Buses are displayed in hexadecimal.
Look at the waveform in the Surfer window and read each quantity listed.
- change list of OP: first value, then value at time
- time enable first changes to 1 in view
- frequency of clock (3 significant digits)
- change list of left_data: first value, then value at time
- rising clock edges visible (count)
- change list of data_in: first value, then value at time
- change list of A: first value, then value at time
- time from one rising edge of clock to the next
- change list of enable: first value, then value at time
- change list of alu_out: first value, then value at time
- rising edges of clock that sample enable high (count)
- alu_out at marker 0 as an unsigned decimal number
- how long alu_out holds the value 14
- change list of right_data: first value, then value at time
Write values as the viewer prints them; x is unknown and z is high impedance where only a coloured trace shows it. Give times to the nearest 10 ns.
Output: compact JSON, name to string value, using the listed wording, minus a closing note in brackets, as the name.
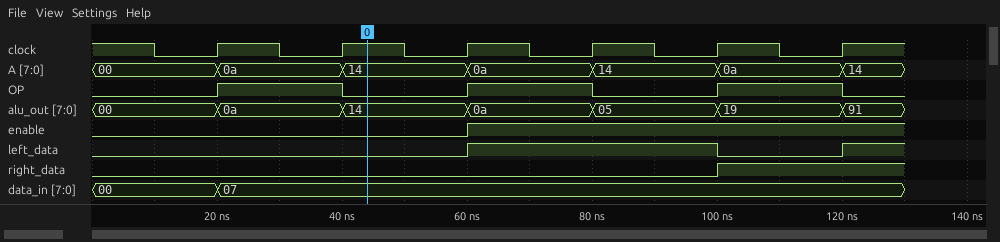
{"change list of OP: first value, then value at time": "0, 1 at 20 ns, 0 at 40 ns, 1 at 60 ns, 0 at 80 ns, 1 at 100 ns, 0 at 120 ns", "time enable first changes to 1 in view": "60 ns", "frequency of clock": "50.0 MHz", "change list of left_data: first value, then value at time": "0, 1 at 60 ns, 0 at 100 ns, 1 at 120 ns", "rising clock edges visible": "6", "change list of data_in: first value, then value at time": "00, 07 at 20 ns", "change list of A: first value, then value at time": "00, 0a at 20 ns, 14 at 40 ns, 0a at 60 ns, 14 at 80 ns, 0a at 100 ns, 14 at 120 ns", "time from one rising edge of clock to the next": "20 ns", "change list of enable: first value, then value at time": "0, 1 at 60 ns", "change list of alu_out: first value, then value at time": "00, 0a at 20 ns, 14 at 40 ns, 0a at 60 ns, 05 at 80 ns, 19 at 100 ns, 91 at 120 ns", "rising edges of clock that sample enable high": "3", "alu_out at marker 0 as an unsigned decimal number": "20", "how long alu_out holds the value 14": "20 ns", "change list of right_data: first value, then value at time": "0, 1 at 100 ns"}
